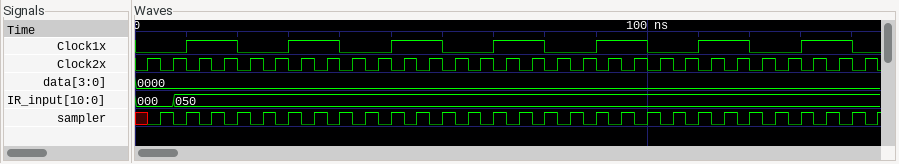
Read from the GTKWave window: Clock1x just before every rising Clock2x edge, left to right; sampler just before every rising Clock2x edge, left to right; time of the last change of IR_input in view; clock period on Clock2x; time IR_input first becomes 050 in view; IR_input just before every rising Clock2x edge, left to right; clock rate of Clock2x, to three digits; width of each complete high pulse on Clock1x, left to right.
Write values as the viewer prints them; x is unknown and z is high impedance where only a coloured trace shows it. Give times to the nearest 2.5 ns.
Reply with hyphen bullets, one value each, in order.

- 0 0 1 1 0 0 1 1 0 0 1 1 0 0 1 1 0 0 1 1 0 0 1 1 0 0 1 1 0
- x 1 1 1 1 1 1 1 1 1 1 1 1 1 1 1 1 1 1 1 1 1 1 1 1 1 1 1 1
- 7.5 ns
- 5 ns
- 7.5 ns
- 000, 000, 050, 050, 050, 050, 050, 050, 050, 050, 050, 050, 050, 050, 050, 050, 050, 050, 050, 050, 050, 050, 050, 050, 050, 050, 050, 050, 050
- 200 MHz
- 10 ns, 10 ns, 10 ns, 10 ns, 10 ns, 10 ns, 10 ns
